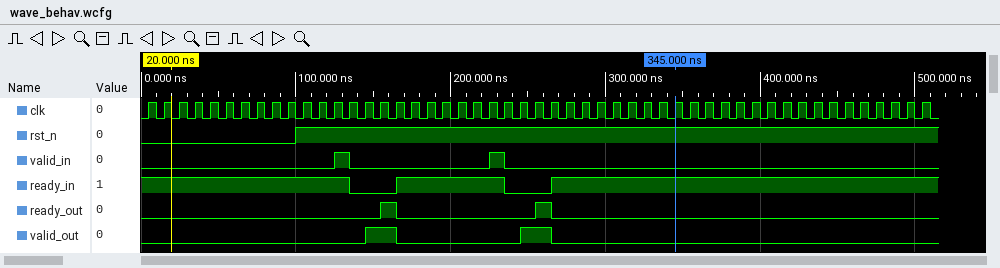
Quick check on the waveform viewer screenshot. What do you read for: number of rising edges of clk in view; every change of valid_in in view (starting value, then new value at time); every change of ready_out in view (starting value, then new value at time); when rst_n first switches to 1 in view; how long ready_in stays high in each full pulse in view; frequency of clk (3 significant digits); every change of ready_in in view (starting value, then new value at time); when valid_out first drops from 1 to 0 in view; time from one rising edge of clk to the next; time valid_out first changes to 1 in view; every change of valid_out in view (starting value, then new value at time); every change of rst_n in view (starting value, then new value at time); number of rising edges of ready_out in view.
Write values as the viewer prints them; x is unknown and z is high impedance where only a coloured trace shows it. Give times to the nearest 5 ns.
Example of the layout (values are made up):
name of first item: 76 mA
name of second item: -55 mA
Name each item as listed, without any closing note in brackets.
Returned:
number of rising edges of clk in view: 51
every change of valid_in in view: 0, 1 at 125 ns, 0 at 135 ns, 1 at 225 ns, 0 at 235 ns
every change of ready_out in view: 0, 1 at 155 ns, 0 at 165 ns, 1 at 255 ns, 0 at 265 ns
when rst_n first switches to 1 in view: 100 ns
how long ready_in stays high in each full pulse in view: 70 ns
frequency of clk: 100 MHz
every change of ready_in in view: 1, 0 at 135 ns, 1 at 165 ns, 0 at 235 ns, 1 at 265 ns
when valid_out first drops from 1 to 0 in view: 165 ns
time from one rising edge of clk to the next: 10 ns
time valid_out first changes to 1 in view: 145 ns
every change of valid_out in view: 0, 1 at 145 ns, 0 at 165 ns, 1 at 245 ns, 0 at 265 ns
every change of rst_n in view: 0, 1 at 100 ns
number of rising edges of ready_out in view: 2
